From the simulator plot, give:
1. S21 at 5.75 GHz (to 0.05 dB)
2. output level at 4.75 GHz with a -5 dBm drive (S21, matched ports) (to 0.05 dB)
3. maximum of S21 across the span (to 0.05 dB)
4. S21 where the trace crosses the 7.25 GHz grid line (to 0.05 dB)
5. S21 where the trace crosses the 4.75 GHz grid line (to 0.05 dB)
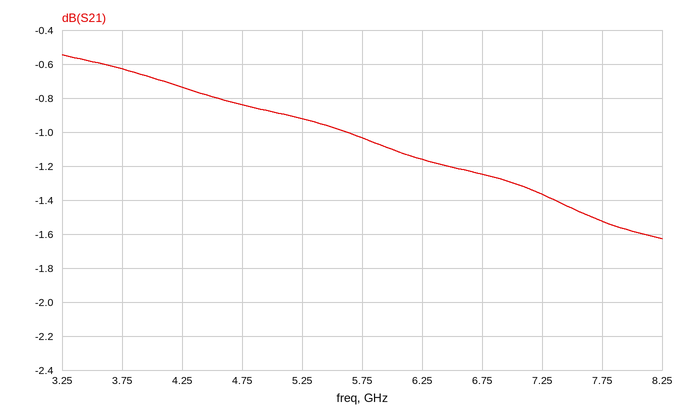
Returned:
-1.05 dB
-5.85 dBm
-0.55 dB
-1.35 dB
-0.85 dB
